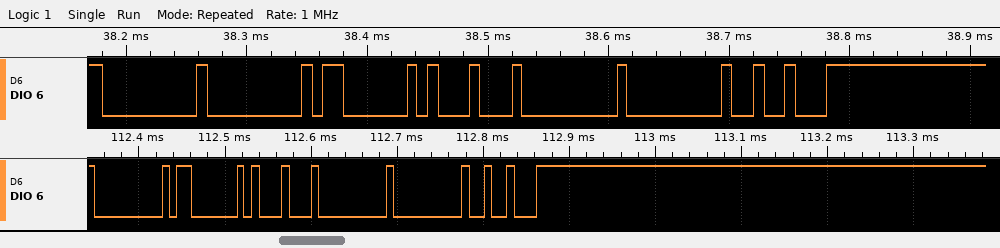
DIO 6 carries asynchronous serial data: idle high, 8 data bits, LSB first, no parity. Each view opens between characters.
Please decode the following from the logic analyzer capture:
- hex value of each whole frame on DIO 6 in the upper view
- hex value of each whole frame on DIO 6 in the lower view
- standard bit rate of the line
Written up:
00, 00, 03, 11, 00, 00, 12
00, 03, 11, 00, 00, 12
115200 baud
